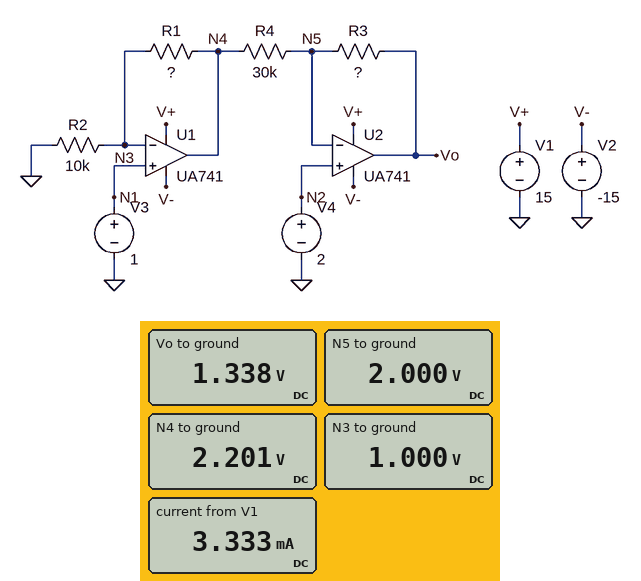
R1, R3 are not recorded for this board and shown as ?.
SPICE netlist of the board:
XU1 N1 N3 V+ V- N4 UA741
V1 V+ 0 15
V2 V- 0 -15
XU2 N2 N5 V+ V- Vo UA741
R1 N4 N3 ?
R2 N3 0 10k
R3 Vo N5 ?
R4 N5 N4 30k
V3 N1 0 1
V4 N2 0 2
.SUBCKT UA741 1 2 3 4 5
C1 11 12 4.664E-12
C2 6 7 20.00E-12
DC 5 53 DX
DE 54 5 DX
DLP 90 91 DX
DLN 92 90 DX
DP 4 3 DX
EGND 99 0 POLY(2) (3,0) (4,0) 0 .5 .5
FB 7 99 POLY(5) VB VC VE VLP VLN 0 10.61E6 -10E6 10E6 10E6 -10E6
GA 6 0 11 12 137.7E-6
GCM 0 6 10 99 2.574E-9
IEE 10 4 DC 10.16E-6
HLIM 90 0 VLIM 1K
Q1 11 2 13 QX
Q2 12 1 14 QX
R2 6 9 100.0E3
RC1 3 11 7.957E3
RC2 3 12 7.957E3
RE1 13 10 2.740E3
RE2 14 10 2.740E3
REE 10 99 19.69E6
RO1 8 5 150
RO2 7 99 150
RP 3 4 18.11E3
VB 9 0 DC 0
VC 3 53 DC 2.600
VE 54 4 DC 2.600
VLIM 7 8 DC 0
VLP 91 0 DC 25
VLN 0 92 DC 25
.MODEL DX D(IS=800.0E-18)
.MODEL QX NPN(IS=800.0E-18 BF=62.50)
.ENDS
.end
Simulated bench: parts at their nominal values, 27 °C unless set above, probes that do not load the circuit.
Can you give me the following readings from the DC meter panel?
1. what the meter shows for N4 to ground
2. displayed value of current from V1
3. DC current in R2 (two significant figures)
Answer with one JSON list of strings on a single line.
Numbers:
["2.201 V", "3.333 mA", "100 µA"]
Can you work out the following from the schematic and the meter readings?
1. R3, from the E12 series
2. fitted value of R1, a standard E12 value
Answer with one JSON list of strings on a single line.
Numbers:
["100 kΩ", "12 kΩ"]
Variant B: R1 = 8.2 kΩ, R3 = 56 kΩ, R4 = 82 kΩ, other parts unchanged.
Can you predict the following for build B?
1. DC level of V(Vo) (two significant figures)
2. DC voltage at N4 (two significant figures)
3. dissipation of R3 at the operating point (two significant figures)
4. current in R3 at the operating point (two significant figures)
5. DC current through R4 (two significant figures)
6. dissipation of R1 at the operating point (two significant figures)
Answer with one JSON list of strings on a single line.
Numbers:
["2.1 V", "1.8 V", "290 nW", "2.3 µA", "2.2 µA", "82 µW"]
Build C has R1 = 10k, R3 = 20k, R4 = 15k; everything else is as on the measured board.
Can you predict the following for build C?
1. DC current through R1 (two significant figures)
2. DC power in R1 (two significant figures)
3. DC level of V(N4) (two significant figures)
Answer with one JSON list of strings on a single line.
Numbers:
["100 µA", "100 µW", "2.0 V"]
